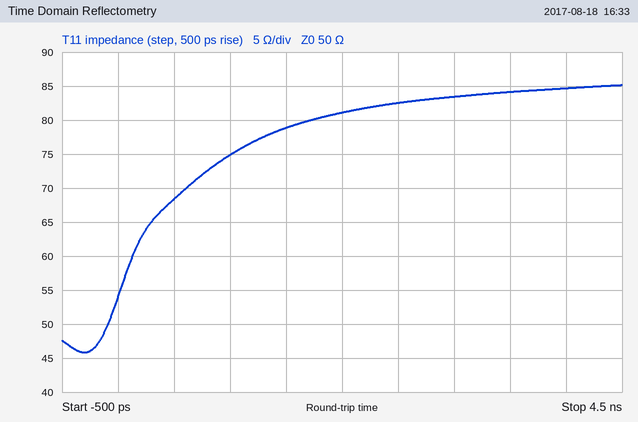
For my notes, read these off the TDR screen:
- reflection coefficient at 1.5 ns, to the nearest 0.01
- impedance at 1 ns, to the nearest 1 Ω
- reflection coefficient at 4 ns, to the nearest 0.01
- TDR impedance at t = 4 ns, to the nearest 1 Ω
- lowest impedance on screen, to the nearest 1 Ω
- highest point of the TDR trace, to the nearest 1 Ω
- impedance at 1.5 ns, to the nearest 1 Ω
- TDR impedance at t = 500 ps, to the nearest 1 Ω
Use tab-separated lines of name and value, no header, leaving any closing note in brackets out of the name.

reflection coefficient at 1.5 ns, to the nearest 0.01	+0.22
impedance at 1 ns, to the nearest 1 Ω	75 Ω
reflection coefficient at 4 ns, to the nearest 0.01	+0.26
TDR impedance at t = 4 ns, to the nearest 1 Ω	85 Ω
lowest impedance on screen, to the nearest 1 Ω	46 Ω
highest point of the TDR trace, to the nearest 1 Ω	85 Ω
impedance at 1.5 ns, to the nearest 1 Ω	79 Ω
TDR impedance at t = 500 ps, to the nearest 1 Ω	68 Ω
